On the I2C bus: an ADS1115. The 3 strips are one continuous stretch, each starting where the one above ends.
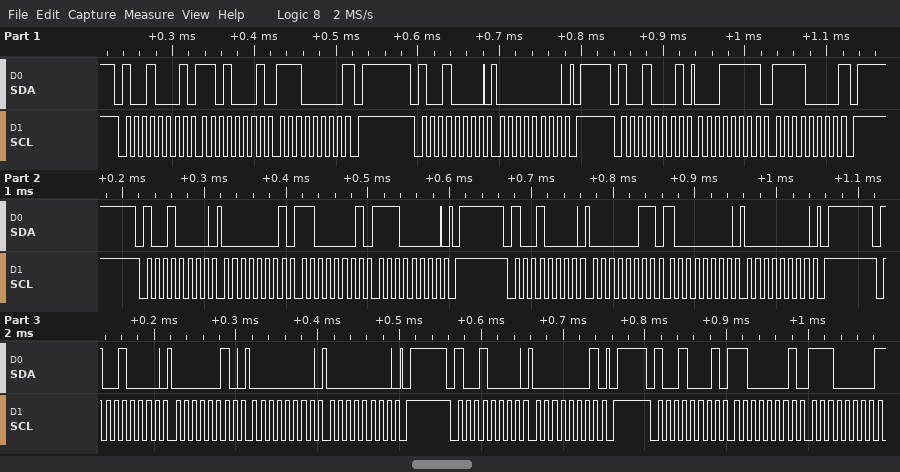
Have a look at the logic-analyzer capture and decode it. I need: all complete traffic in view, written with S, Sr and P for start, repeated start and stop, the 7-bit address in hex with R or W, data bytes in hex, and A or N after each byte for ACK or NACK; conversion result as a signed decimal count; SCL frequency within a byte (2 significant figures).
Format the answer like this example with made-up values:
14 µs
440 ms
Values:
S 48R A D1 A E0 N P S 48W A 00 A P S 48R A 1F A F0 N P S 48W A 01 A C1 A E0 A P S 48W A 03 A 80 A 00 A P S 48W A 02 A 00 A 00 A P S 48W A 01 A P S 48R A C1 A E0 N
8176
100 kHz
